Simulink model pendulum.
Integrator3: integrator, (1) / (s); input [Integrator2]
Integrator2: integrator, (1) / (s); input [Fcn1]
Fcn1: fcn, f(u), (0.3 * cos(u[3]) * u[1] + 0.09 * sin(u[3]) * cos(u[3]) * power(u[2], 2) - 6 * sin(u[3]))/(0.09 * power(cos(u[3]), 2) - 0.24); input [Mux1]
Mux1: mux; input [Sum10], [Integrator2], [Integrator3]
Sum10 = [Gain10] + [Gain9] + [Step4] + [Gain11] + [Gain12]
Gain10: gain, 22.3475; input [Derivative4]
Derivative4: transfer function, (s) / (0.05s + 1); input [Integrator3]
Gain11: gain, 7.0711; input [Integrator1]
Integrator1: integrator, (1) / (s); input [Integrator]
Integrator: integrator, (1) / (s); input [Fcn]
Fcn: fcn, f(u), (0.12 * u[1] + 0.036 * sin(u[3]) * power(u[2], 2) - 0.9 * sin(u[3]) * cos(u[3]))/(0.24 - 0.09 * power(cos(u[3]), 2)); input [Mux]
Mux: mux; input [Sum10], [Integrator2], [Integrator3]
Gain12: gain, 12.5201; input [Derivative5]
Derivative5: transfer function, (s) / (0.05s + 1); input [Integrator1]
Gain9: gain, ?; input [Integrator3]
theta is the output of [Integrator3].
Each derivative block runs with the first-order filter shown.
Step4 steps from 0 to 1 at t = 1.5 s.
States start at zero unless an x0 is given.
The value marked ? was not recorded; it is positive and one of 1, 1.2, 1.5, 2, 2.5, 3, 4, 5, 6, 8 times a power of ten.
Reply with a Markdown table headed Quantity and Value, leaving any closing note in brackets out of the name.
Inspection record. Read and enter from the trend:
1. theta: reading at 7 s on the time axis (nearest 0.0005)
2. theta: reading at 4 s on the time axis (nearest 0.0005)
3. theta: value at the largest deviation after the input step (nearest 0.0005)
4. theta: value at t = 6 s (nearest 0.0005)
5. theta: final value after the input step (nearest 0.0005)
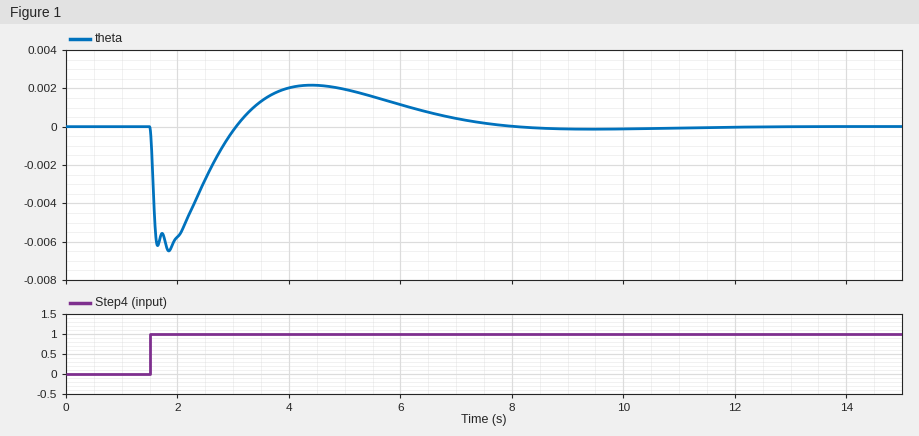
| Quantity | Value |
|---|---|
| theta: reading at 7 s on the time axis | 0.0005 |
| theta: reading at 4 s on the time axis | 0.0020 |
| theta: value at the largest deviation after the input step | -0.0065 |
| theta: value at t = 6 s | 0.0010 |
| theta: final value after the input step | 0.0000 |
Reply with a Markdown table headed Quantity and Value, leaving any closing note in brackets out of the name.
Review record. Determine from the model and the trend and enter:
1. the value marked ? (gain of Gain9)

| Quantity | Value |
|---|---|
| the value marked ? | 150 |
